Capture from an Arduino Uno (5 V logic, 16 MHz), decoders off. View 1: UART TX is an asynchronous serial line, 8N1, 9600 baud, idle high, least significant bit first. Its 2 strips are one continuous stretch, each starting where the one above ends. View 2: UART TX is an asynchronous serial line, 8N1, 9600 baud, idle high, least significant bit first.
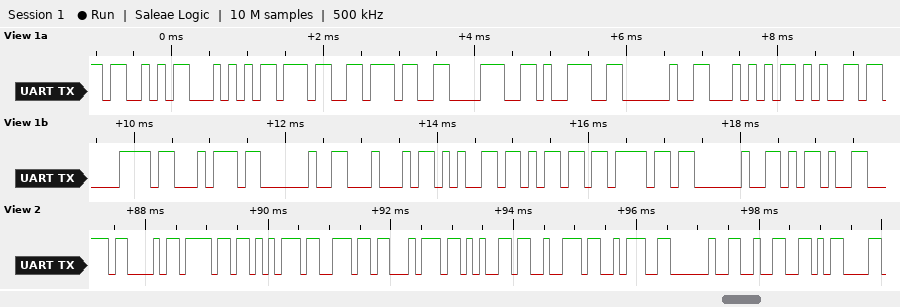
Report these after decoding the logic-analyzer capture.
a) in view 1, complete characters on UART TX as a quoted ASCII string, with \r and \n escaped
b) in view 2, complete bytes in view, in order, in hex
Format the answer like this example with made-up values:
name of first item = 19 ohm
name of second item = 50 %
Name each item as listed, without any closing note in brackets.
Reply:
in view 1, complete characters on UART TX as a quoted ASCII string, with \r and \n escaped = "ST7789 Text Demo -"
in view 2, complete bytes in view, in order, in hex = 43 6F 75 6E 74 65 72 3A 20 32 0D
